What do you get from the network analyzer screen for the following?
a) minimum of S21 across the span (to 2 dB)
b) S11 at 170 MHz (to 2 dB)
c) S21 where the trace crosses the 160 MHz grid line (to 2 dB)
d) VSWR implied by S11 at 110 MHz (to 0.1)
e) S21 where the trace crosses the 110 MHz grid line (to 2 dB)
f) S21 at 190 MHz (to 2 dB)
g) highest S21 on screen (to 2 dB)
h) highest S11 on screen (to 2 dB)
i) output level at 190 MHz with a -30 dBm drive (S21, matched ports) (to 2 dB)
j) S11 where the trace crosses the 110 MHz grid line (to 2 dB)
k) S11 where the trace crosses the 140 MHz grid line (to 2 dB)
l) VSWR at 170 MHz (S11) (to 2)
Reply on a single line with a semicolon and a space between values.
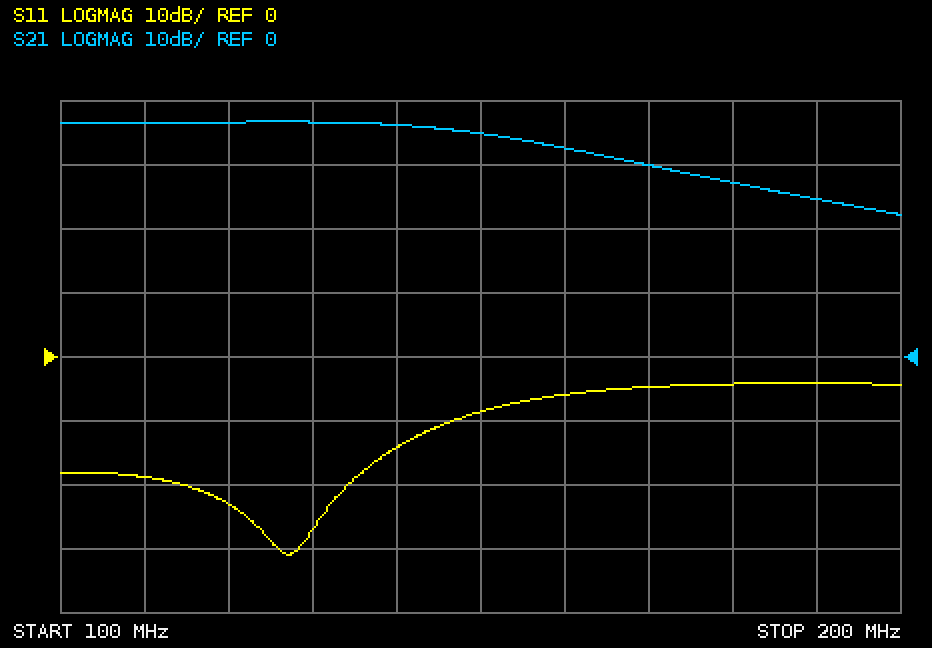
22 dB; -4 dB; 32 dB; 1.3; 36 dB; 24 dB; 36 dB; -4 dB; -6 dBm; -18 dB; -14 dB; 4
